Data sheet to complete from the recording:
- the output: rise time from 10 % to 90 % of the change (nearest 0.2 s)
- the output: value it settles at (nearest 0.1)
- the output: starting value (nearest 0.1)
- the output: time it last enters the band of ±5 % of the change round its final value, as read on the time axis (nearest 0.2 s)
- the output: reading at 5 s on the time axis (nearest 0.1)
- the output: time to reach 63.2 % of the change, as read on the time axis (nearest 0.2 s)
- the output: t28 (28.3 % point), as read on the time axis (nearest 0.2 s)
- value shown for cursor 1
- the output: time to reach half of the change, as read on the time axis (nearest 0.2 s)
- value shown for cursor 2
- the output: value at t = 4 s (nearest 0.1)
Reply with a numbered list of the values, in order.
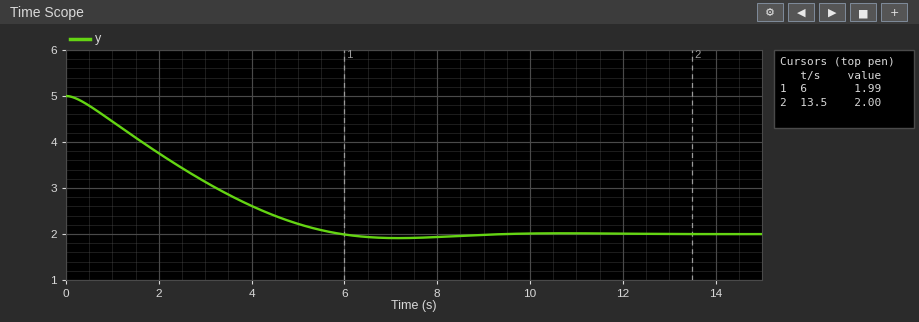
1. 4.2 s
2. 2.0
3. 5.0
4. 5.2 s
5. 2.2
6. 3.0 s
7. 1.4 s
8. 1.99
9. 2.4 s
10. 2.00
11. 2.6
